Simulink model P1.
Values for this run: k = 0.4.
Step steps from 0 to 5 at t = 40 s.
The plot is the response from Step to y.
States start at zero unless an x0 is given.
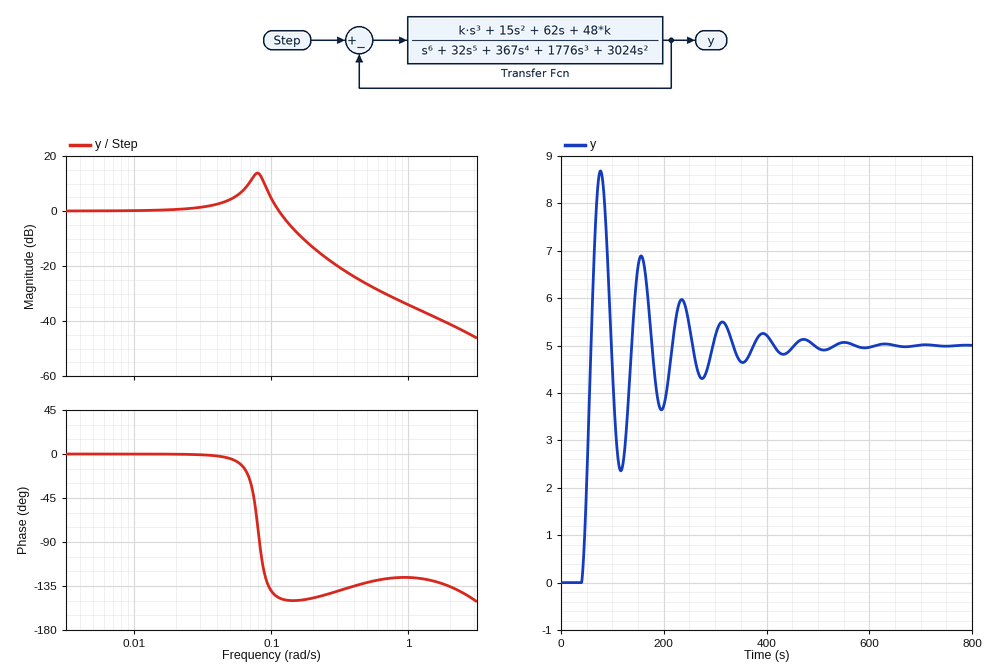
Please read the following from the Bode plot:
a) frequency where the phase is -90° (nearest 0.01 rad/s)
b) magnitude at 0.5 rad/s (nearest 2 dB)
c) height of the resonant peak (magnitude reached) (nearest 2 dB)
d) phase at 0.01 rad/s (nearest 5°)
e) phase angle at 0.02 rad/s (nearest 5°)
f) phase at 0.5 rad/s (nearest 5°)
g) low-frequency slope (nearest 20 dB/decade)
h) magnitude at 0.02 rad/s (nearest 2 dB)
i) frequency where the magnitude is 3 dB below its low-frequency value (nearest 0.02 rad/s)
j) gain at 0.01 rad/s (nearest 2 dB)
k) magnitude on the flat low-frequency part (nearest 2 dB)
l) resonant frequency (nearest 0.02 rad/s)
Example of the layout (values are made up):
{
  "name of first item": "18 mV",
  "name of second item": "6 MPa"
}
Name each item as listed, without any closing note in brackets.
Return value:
{
  "frequency where the phase is -90°": "0.08 rad/s",
  "magnitude at 0.5 rad/s": "-26 dB",
  "height of the resonant peak (magnitude reached)": "14 dB",
  "phase at 0.01 rad/s": "0°",
  "phase angle at 0.02 rad/s": "0°",
  "phase at 0.5 rad/s": "-130°",
  "low-frequency slope": "0 dB/decade",
  "magnitude at 0.02 rad/s": "0 dB",
  "frequency where the magnitude is 3 dB below its low-frequency value": "0.12 rad/s",
  "gain at 0.01 rad/s": "0 dB",
  "magnitude on the flat low-frequency part": "0 dB",
  "resonant frequency": "0.08 rad/s"
}
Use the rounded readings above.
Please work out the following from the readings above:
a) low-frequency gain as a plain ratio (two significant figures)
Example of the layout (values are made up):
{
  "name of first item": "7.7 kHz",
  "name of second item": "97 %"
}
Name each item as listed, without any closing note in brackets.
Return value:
{
  "low-frequency gain as a plain ratio": "1.0"
}
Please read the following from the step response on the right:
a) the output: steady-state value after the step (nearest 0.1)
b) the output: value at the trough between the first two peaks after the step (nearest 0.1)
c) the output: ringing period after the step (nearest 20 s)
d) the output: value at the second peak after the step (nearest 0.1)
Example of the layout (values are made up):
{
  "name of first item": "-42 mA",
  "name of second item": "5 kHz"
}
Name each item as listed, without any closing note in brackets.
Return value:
{
  "the output: steady-state value after the step": "5.0",
  "the output: value at the trough between the first two peaks after the step": "2.4",
  "the output: ringing period after the step": "80 s",
  "the output: value at the second peak after the step": "6.9"
}
